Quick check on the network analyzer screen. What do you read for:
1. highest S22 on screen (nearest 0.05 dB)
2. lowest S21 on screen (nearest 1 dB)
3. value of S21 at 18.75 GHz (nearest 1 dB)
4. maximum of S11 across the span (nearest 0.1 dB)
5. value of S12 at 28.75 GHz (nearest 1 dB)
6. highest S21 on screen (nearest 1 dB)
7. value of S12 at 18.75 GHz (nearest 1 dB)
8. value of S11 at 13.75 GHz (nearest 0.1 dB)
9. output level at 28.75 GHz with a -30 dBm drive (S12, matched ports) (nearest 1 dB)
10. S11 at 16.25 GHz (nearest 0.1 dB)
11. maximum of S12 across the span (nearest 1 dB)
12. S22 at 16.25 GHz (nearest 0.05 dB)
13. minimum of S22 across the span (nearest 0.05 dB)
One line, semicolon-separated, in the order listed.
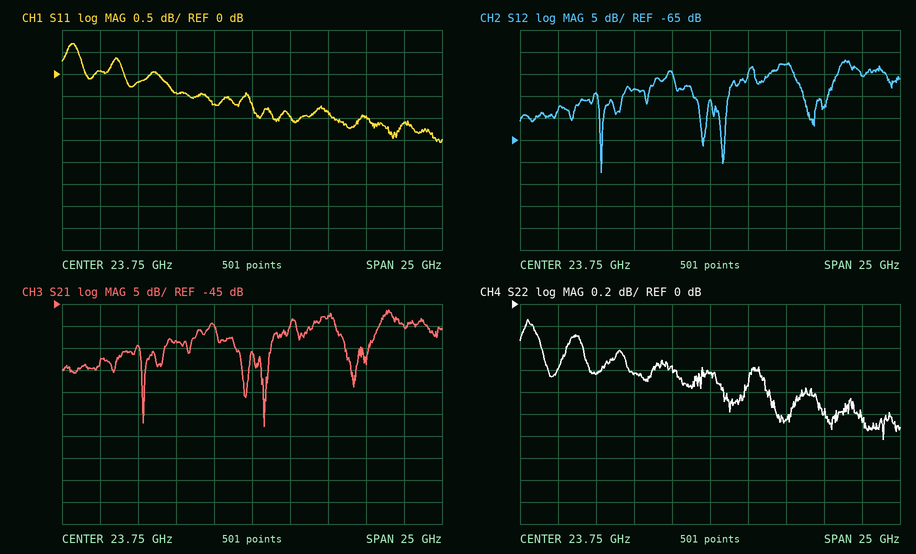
-0.15 dB; -73 dB; -53 dB; 0.7 dB; -48 dB; -46 dB; -53 dB; 0.1 dB; -78 dBm; -0.2 dB; -47 dB; -0.65 dB; -1.25 dB
